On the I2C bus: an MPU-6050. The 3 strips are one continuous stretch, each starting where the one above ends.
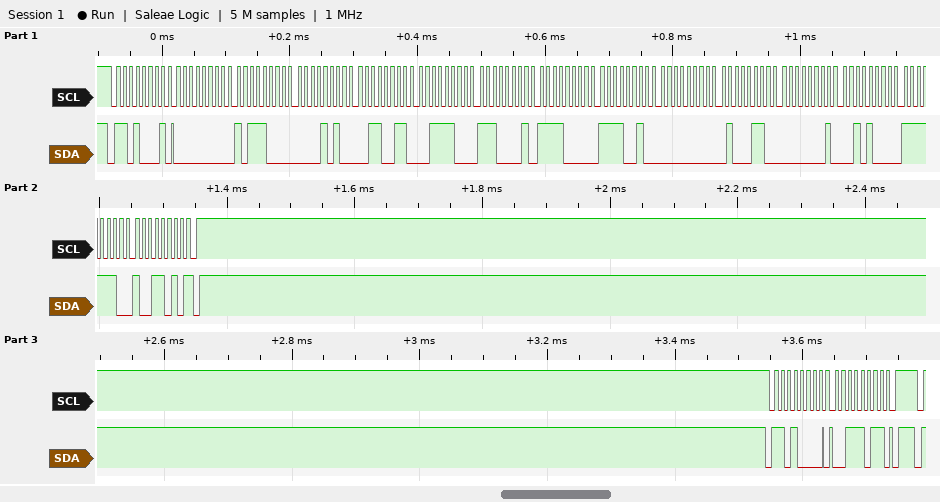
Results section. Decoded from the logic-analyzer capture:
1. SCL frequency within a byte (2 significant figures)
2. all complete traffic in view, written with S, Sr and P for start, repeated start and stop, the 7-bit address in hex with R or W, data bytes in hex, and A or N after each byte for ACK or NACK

100 kHz
S 68R A 00 A B8 A 0A A 33 A 3C A E1 A F0 A F2 A 00 A 46 A 01 A 28 A FE A 9A N P S 68W A 3B A P
